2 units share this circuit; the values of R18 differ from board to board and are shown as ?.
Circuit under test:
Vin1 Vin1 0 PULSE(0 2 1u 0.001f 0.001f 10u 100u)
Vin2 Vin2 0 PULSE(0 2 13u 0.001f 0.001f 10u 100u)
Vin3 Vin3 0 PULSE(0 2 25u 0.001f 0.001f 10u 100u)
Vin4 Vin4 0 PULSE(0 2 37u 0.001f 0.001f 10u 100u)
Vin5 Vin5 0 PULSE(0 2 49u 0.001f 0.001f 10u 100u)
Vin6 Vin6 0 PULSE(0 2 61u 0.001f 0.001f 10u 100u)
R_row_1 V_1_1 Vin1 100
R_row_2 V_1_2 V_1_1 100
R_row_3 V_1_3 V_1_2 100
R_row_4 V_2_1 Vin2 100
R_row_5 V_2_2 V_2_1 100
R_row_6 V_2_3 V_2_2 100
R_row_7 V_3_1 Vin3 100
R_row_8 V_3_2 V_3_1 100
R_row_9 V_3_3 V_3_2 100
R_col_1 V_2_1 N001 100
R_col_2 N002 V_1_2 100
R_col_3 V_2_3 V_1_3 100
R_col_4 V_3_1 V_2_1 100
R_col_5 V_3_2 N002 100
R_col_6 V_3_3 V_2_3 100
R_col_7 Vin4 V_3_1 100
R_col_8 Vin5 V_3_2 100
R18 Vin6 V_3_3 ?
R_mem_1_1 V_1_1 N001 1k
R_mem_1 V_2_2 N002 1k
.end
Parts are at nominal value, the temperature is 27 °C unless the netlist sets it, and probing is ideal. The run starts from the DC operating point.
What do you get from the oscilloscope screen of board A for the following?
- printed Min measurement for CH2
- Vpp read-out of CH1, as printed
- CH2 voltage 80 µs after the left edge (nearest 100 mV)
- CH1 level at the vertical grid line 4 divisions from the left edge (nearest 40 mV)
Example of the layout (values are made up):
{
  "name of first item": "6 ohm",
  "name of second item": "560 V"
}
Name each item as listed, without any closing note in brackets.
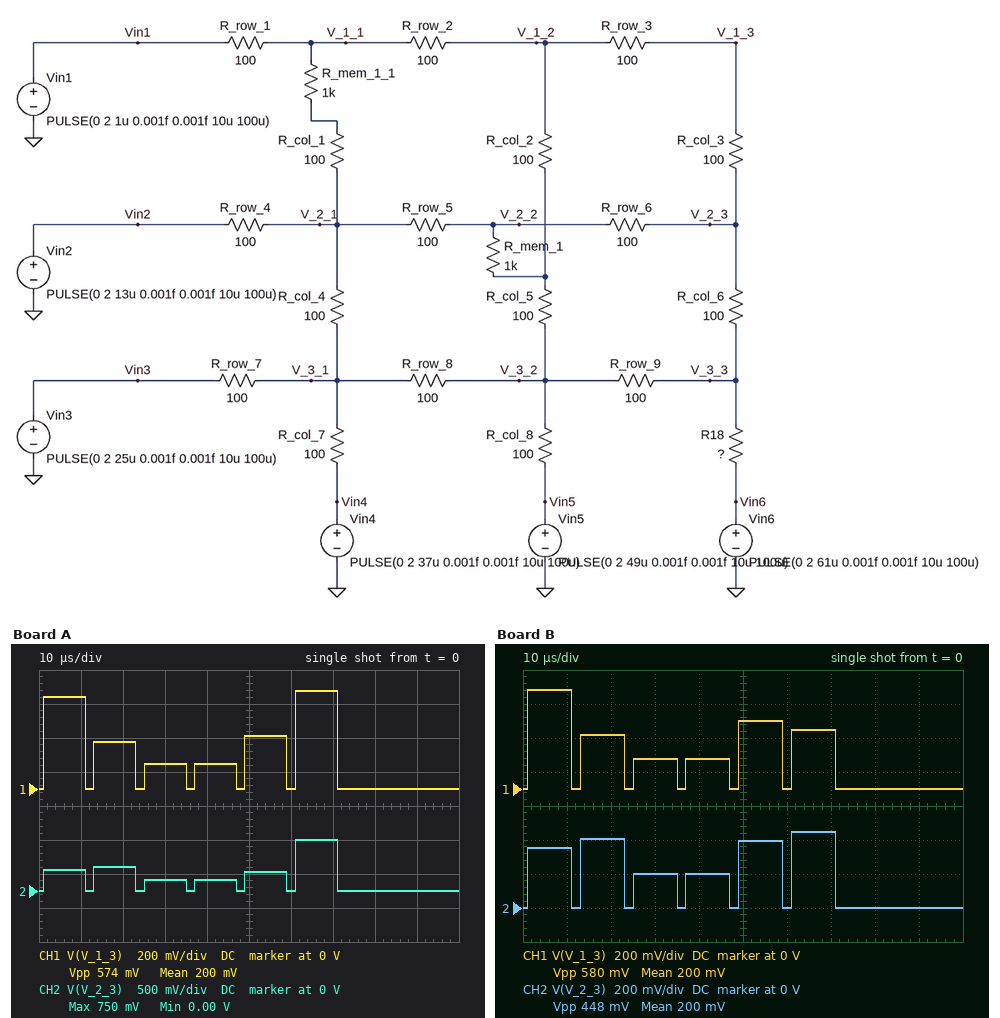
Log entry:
{
  "printed Min measurement for CH2": "0.00 V",
  "Vpp read-out of CH1, as printed": "574 mV",
  "CH2 voltage 80 µs after the left edge": "0 V",
  "CH1 level at the vertical grid line 4 divisions from the left edge": "160 mV"
}
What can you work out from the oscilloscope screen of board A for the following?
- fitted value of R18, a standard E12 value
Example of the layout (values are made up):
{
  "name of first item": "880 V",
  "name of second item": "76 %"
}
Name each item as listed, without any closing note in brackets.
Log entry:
{
  "fitted value of R18, a standard E12 value": "68 Ω"
}
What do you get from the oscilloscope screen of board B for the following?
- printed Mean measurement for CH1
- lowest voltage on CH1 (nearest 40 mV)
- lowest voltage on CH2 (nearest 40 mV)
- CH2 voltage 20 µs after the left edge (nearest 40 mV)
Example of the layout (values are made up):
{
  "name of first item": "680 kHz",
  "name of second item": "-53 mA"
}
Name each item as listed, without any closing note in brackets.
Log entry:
{
  "printed Mean measurement for CH1": "200 mV",
  "lowest voltage on CH1": "0 V",
  "lowest voltage on CH2": "0 V",
  "CH2 voltage 20 µs after the left edge": "400 mV"
}
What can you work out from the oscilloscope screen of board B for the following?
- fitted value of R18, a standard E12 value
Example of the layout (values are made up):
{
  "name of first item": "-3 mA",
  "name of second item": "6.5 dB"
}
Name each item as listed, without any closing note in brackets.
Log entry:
{
  "fitted value of R18, a standard E12 value": "180 Ω"
}
